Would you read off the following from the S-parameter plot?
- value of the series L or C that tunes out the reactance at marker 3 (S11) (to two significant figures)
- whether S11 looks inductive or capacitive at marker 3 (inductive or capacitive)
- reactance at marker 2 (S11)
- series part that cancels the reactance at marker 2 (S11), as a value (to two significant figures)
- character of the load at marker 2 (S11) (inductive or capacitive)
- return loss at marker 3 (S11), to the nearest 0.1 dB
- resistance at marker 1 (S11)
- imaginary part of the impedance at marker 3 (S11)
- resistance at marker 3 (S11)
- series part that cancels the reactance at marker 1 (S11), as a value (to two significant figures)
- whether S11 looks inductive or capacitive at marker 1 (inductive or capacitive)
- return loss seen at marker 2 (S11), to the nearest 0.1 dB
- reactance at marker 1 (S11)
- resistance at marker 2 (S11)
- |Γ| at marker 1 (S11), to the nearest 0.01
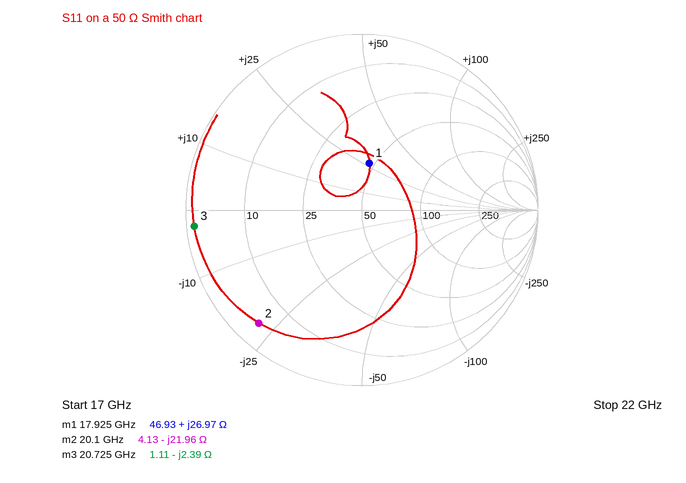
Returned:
18 pH
capacitive
-21.96 Ω
170 pH
capacitive
0.4 dB
46.93 Ω
-2.39 Ω
1.11 Ω
330 fF
inductive
1.2 dB
+26.97 Ω
4.13 Ω
0.27
